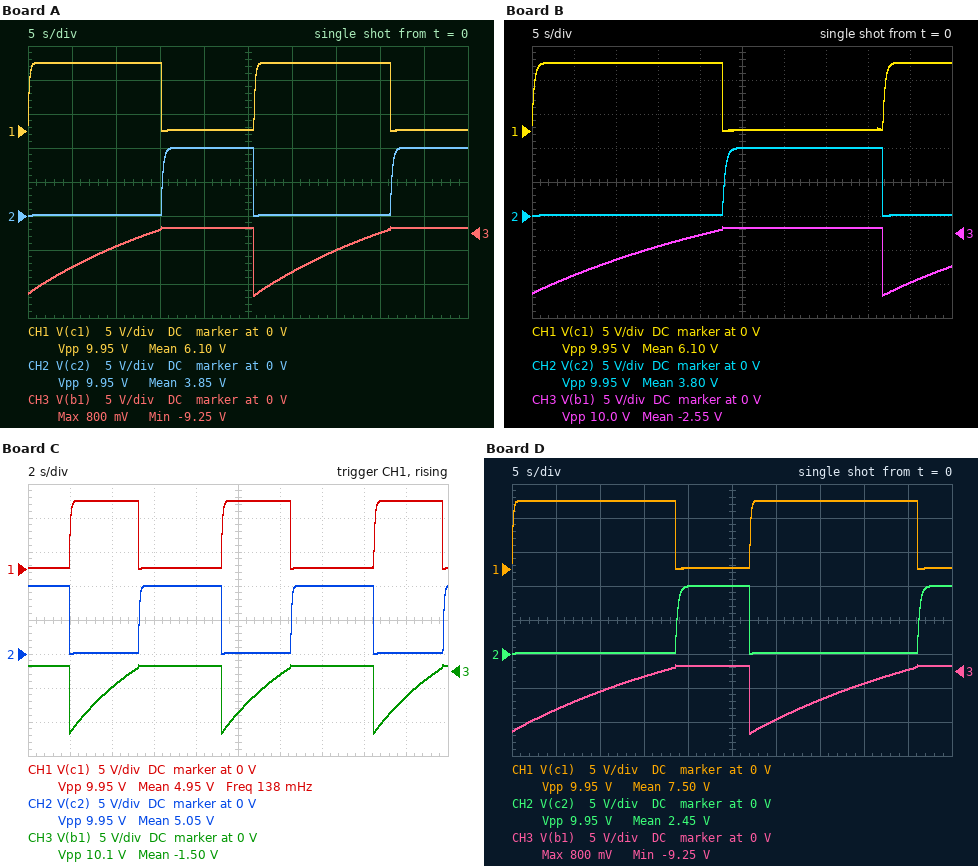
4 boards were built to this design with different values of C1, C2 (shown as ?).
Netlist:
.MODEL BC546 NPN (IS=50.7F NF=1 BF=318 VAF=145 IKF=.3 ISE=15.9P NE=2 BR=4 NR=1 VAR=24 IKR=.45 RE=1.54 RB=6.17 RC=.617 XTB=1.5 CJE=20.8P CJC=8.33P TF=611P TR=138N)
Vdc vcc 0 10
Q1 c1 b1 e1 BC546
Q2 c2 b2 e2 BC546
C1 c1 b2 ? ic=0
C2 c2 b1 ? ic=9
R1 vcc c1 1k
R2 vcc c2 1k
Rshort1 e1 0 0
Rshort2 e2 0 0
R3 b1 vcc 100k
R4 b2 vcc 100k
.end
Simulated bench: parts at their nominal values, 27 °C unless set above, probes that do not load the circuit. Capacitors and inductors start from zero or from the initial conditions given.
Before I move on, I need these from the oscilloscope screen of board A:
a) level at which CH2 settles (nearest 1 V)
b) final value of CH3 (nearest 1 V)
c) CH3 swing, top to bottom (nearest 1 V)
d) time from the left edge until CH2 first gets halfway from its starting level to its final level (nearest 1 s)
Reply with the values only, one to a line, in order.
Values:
10 V
1 V
10 V
15 s
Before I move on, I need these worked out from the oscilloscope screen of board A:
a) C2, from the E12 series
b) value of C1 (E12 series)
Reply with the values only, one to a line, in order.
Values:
220 µF
150 µF
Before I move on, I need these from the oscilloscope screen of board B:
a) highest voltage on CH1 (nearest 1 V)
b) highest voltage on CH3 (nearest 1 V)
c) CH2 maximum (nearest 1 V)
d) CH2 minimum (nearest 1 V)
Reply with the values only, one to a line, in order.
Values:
10 V
1 V
10 V
0 V
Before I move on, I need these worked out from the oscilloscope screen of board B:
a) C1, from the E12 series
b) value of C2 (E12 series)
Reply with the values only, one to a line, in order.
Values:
270 µF
330 µF
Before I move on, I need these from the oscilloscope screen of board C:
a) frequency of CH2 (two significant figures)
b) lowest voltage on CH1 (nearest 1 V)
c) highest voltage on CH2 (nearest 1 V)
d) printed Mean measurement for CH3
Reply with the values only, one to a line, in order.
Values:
140 mHz
0 V
10 V
-1.50 V
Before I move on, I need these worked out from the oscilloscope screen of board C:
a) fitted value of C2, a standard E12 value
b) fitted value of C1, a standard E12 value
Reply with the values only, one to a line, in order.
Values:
47 µF
56 µF
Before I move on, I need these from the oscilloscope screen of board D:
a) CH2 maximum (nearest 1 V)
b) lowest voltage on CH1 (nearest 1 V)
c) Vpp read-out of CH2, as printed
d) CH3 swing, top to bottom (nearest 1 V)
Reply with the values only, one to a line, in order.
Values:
10 V
0 V
9.95 V
10 V
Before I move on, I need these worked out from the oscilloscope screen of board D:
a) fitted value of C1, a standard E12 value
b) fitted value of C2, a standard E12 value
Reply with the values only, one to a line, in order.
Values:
120 µF
270 µF
